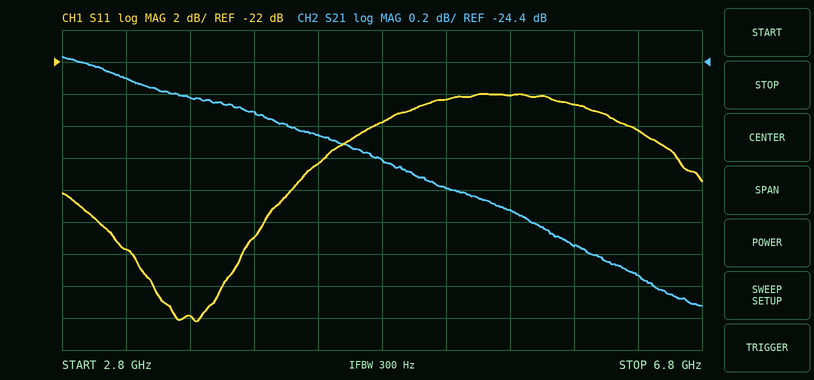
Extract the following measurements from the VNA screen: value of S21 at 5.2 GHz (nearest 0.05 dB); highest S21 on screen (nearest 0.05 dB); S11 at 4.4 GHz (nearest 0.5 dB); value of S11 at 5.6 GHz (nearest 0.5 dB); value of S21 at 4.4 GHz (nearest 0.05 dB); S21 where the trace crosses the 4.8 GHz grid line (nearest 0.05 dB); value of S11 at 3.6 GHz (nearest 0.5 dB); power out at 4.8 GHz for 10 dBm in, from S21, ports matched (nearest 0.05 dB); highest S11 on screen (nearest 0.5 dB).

-25.20 dB
-24.35 dB
-28.5 dB
-24.0 dB
-24.85 dB
-25.00 dB
-38.0 dB
-15.00 dBm
-24.0 dB
